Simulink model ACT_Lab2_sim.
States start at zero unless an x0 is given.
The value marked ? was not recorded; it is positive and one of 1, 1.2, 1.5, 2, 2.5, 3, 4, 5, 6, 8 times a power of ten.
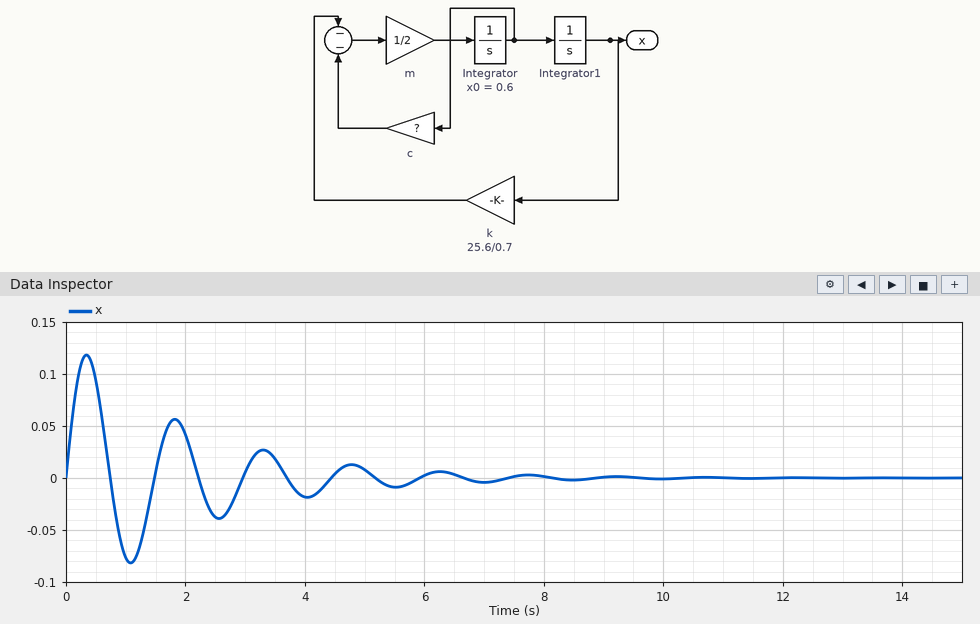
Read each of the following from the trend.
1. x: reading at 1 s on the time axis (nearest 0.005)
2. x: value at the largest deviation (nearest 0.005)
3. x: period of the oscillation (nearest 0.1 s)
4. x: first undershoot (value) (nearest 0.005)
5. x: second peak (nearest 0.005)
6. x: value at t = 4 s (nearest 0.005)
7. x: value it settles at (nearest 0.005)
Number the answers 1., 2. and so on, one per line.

1. -0.075
2. 0.120
3. 1.5 s
4. -0.080
5. 0.055
6. -0.020
7. 0.000
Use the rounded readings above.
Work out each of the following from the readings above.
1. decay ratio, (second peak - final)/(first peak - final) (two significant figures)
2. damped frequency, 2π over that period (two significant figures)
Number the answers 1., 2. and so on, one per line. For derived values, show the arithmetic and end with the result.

1. (0.055 - 0) / (0.12 - 0) = 0.46
2. 2π / 1.5 = 4.2 rad/s
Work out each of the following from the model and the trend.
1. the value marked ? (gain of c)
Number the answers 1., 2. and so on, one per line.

1. 2
